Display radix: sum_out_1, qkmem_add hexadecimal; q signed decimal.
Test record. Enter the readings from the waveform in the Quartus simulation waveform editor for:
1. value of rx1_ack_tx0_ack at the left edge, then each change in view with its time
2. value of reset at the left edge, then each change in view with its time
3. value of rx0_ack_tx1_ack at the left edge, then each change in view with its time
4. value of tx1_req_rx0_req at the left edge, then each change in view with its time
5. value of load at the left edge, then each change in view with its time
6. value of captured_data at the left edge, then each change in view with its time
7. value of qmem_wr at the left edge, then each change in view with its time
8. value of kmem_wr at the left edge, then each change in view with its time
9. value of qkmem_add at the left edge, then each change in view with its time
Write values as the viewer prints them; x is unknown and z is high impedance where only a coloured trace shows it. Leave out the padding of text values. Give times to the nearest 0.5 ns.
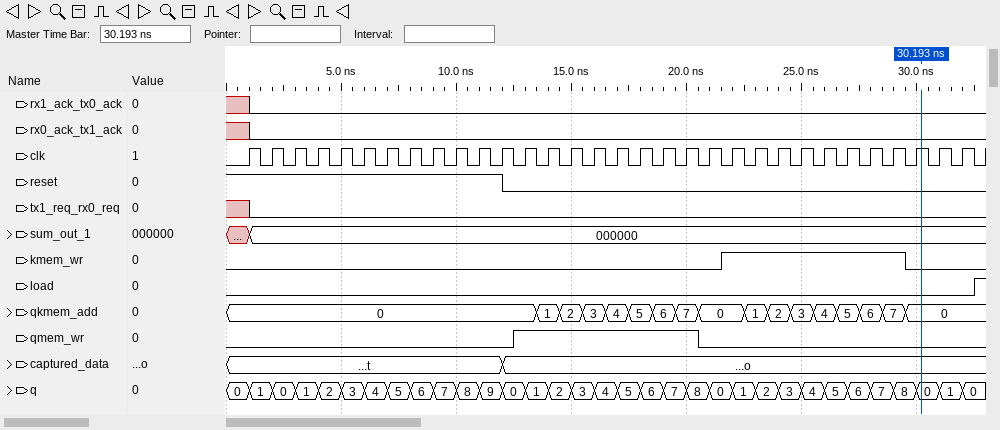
x, 0 at 1 ns
1, 0 at 12 ns
x, 0 at 1 ns
x, 0 at 1 ns
0, 1 at 32.5 ns
t, o at 12 ns
0, 1 at 12.5 ns, 0 at 20.5 ns
0, 1 at 21.5 ns, 0 at 29.5 ns
0, 1 at 13.5 ns, 2 at 14.5 ns, 3 at 15.5 ns, 4 at 16.5 ns, 5 at 17.5 ns, 6 at 18.5 ns, 7 at 19.5 ns, 0 at 20.5 ns, 1 at 22.5 ns, 2 at 23.5 ns, 3 at 24.5 ns, 4 at 25.5 ns, 5 at 26.5 ns, 6 at 27.5 ns, 7 at 28.5 ns, 0 at 29.5 ns
